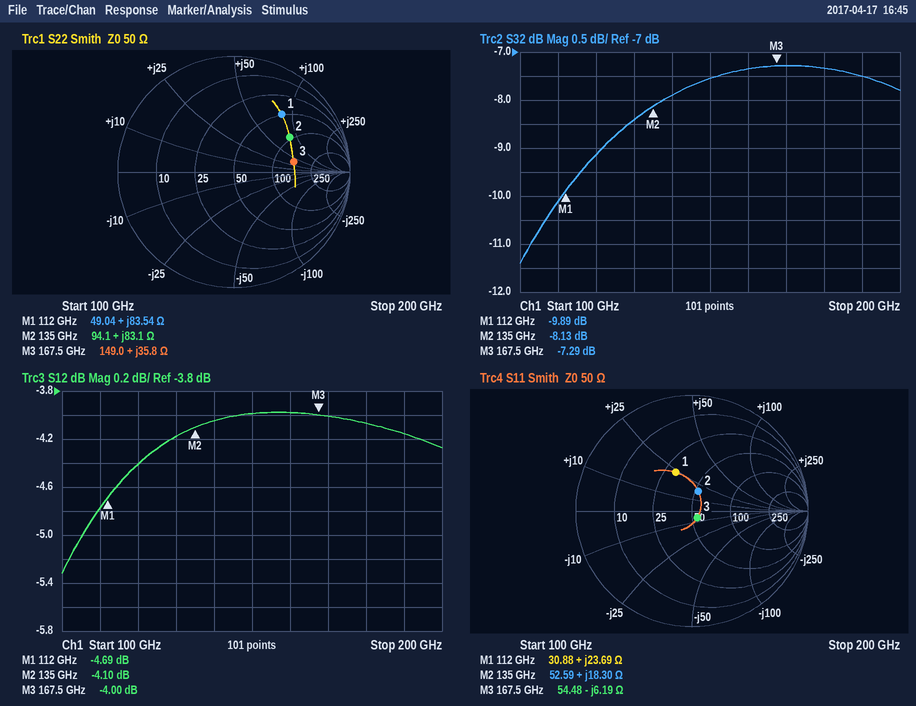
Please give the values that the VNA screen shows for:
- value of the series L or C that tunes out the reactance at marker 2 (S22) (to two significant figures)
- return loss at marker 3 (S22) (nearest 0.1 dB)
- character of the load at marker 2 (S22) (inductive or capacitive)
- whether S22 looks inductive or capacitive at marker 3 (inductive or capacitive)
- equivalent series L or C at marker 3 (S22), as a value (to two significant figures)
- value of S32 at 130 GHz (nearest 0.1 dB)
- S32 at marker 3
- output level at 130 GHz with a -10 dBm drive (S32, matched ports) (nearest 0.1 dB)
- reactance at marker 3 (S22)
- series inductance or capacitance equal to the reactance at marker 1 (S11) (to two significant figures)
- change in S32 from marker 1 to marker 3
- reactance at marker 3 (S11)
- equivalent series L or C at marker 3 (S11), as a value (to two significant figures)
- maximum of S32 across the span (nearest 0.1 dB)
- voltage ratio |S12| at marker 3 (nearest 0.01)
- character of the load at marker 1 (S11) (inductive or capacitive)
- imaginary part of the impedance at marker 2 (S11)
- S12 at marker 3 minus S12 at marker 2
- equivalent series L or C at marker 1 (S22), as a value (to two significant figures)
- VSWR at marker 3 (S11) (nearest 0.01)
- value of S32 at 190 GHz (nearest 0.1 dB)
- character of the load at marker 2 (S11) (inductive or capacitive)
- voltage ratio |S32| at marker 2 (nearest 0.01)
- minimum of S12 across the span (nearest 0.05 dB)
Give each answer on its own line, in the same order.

14 fF
5.7 dB
inductive
inductive
34 pH
-8.4 dB
-7.29 dB
-18.4 dBm
+35.8 Ω
34 pH
2.60 dB
-6.19 Ω
150 fF
-7.3 dB
0.63
inductive
+18.30 Ω
0.10 dB
120 pH
1.16
-7.5 dB
inductive
0.39
-5.30 dB
